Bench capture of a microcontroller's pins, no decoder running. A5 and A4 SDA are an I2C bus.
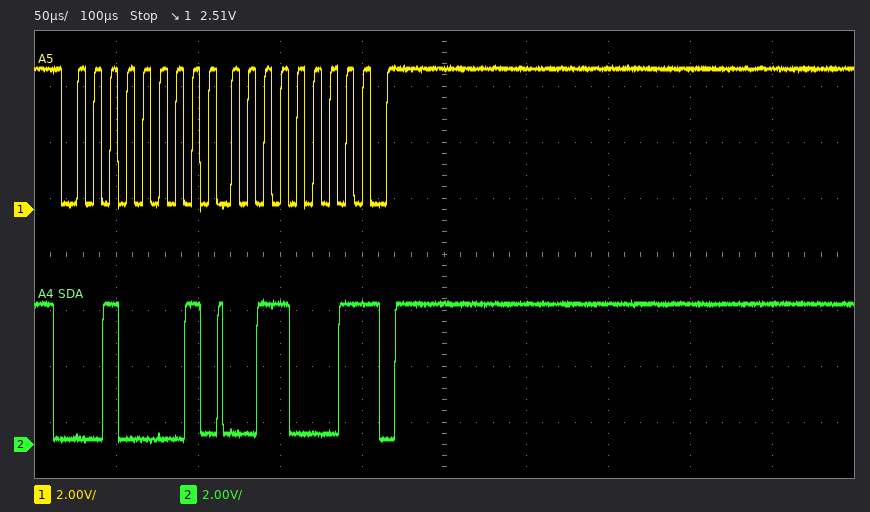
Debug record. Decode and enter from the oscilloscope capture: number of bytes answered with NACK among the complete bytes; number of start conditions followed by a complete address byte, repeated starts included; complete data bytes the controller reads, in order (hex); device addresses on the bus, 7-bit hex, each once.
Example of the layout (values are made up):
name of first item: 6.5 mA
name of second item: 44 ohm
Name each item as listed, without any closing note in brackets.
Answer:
number of bytes answered with NACK among the complete bytes: 1
number of start conditions followed by a complete address byte, repeated starts included: 1
complete data bytes the controller reads, in order: 31
device addresses on the bus, 7-bit hex, each once: 0x10
